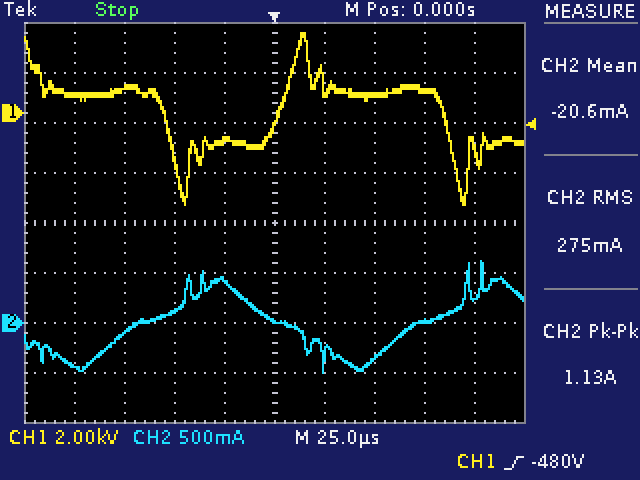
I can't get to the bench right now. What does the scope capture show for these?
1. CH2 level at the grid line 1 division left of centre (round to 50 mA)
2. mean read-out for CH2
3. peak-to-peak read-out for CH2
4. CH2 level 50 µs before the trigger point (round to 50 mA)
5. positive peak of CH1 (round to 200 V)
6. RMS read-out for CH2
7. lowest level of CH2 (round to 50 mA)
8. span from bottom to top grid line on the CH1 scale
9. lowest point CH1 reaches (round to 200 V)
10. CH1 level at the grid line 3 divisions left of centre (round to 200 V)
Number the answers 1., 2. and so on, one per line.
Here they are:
1. 400 mA
2. -20.6 mA
3. 1.13 A
4. 100 mA
5. 3.2 kV
6. 275 mA
7. -500 mA
8. 16 kV
9. -3.6 kV
10. 1.0 kV
